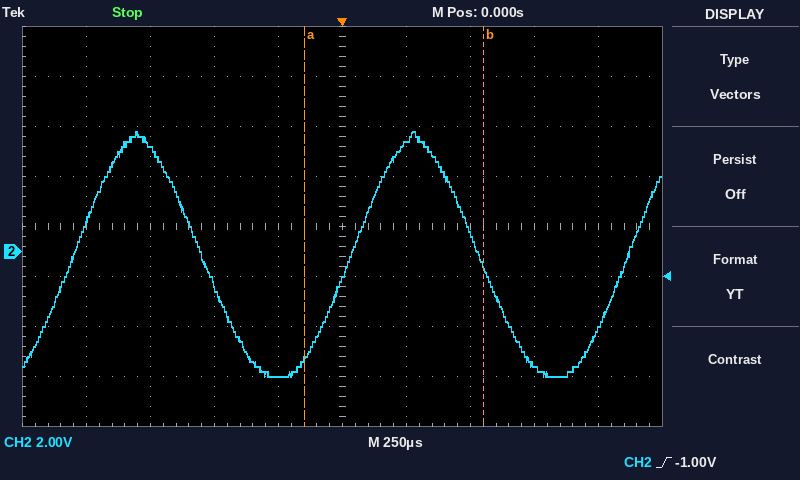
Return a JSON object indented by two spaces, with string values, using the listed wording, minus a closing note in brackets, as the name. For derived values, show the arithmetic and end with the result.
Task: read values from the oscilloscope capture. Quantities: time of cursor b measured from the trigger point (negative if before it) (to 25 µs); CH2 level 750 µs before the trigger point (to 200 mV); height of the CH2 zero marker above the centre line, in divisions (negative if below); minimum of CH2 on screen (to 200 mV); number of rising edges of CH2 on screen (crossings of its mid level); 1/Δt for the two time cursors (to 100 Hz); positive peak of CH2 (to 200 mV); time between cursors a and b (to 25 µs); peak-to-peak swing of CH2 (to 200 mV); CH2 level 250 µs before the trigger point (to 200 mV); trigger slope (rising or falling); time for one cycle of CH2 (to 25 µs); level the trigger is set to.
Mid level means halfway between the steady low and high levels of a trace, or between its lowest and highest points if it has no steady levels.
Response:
{
  "time of cursor b measured from the trigger point (negative if before it)": "+550 µs",
  "CH2 level 750 µs before the trigger point": "4.2 V",
  "height of the CH2 zero marker above the centre line, in divisions": "-0.5 div",
  "minimum of CH2 on screen": "-5.0 V",
  "number of rising edges of CH2 on screen": "3",
  "1/Δt for the two time cursors": "1 / 700 µs ≈ 1.4 kHz",
  "positive peak of CH2": "4.8 V",
  "time between cursors a and b": "700 µs",
  "peak-to-peak swing of CH2": "4.8 V − (-5.0 V) = 9.8 V",
  "CH2 level 250 µs before the trigger point": "-5.0 V",
  "trigger slope": "rising",
  "time for one cycle of CH2": "1.075 ms",
  "level the trigger is set to": "-1.00 V"
}
